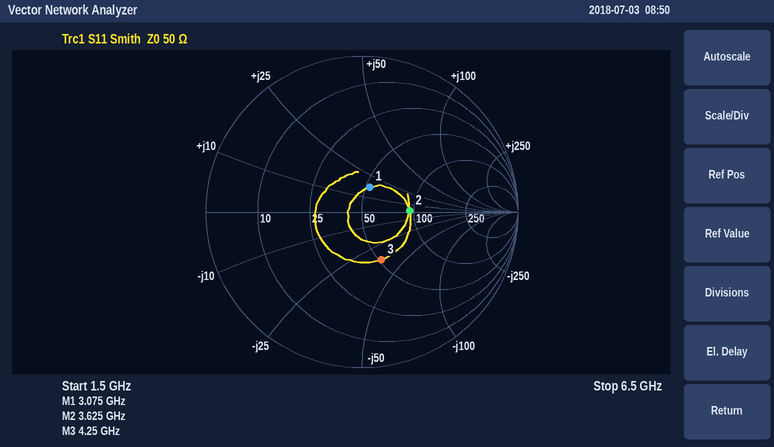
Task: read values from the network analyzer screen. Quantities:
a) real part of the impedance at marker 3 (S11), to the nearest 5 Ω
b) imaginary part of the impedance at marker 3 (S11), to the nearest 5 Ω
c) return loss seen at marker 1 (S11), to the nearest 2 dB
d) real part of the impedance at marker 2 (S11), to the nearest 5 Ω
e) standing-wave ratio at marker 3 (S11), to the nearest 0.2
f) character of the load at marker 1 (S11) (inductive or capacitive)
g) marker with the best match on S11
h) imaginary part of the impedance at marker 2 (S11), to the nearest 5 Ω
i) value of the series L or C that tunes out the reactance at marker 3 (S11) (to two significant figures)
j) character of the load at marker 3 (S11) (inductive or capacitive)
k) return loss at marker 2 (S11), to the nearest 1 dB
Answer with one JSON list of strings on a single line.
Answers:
["50 Ω", "-35 Ω", "16 dB", "95 Ω", "2.0", "inductive", "marker 1", "0 Ω", "1.3 nH", "capacitive", "10 dB"]
